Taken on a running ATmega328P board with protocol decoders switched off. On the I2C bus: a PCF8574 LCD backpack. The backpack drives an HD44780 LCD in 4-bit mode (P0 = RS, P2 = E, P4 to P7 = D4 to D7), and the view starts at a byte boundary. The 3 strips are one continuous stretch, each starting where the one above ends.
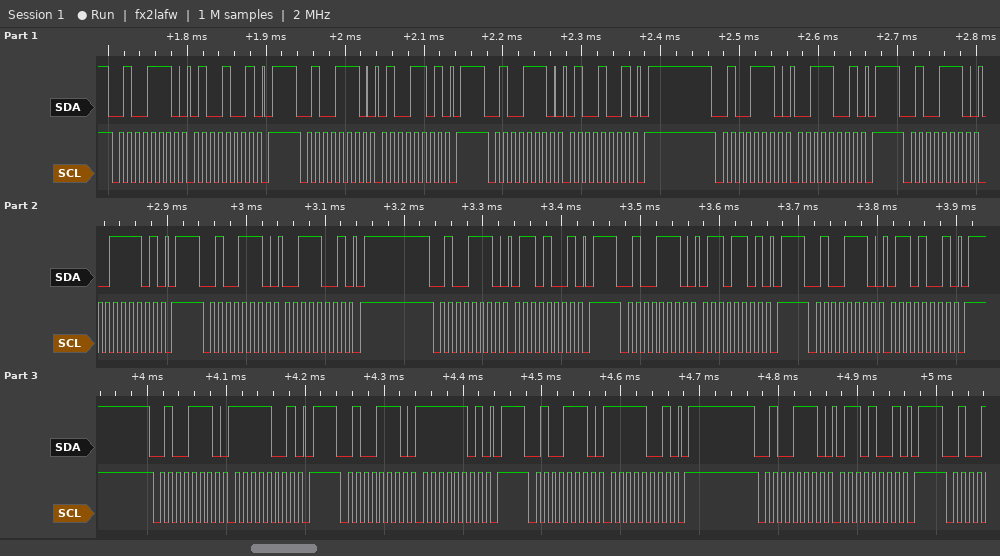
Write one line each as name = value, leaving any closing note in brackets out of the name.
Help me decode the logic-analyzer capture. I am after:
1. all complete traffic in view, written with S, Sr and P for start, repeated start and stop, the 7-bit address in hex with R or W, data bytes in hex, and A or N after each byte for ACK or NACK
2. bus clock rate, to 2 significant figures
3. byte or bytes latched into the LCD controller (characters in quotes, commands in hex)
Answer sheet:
all complete traffic in view, written with S, Sr and P for start, repeated start and stop, the 7-bit address in hex with R or W, data bytes in hex, and A or N after each byte for ACK or NACK = S 27W A 49 A P S 27W A 4D A P S 27W A 49 A P S 27W A 39 A P S 27W A 3D A P S 27W A 39 A P S 27W A 69 A P S 27W A 6D A P S 27W A 69 A P S 27W A F9 A P S 27W A FD A P S 27W A F9 A P S 27W A 69 A P
bus clock rate, to 2 significant figures = 100 kHz
byte or bytes latched into the LCD controller = 'C' 'o'
